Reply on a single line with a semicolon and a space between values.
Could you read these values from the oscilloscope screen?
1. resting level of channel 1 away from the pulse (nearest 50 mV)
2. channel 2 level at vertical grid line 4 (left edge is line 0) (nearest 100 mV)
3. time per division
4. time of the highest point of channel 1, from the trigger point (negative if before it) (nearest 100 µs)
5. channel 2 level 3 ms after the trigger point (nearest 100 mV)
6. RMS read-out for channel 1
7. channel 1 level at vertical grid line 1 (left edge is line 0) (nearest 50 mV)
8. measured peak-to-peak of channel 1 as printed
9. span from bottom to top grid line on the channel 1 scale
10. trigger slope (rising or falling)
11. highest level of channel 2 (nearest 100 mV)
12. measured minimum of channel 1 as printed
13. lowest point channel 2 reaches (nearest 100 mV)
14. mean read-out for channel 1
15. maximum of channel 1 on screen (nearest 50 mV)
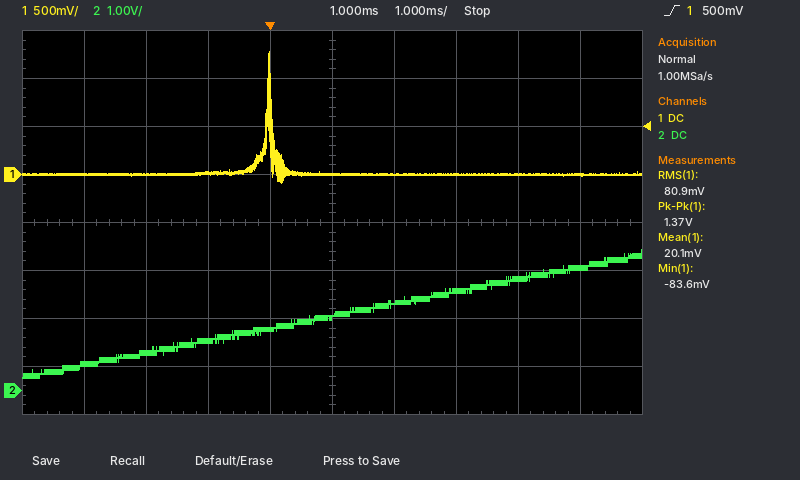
0 mV; 1.3 V; 1 ms; 0.0 ms; 2.1 V; 80.9 mV; 0 mV; 1.37 V; 4 V; rising; 2.9 V; -83.6 mV; 300 mV; 20.1 mV; 1.30 V
